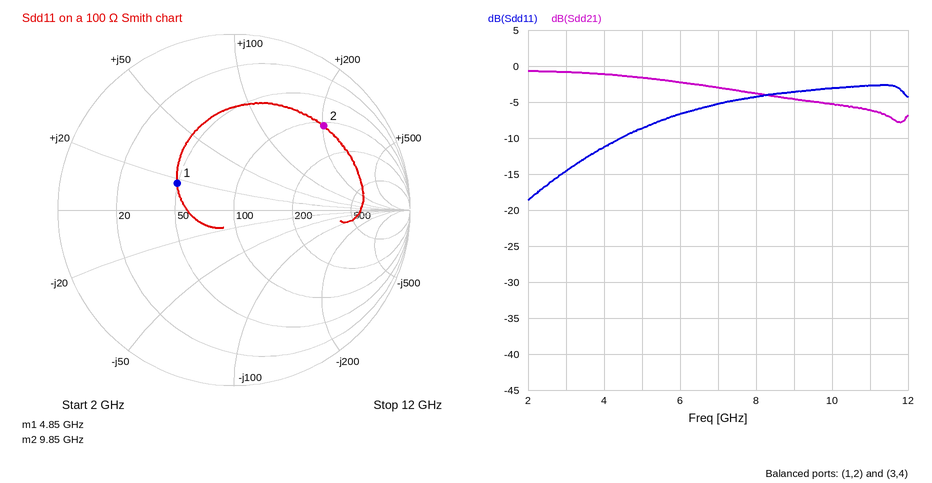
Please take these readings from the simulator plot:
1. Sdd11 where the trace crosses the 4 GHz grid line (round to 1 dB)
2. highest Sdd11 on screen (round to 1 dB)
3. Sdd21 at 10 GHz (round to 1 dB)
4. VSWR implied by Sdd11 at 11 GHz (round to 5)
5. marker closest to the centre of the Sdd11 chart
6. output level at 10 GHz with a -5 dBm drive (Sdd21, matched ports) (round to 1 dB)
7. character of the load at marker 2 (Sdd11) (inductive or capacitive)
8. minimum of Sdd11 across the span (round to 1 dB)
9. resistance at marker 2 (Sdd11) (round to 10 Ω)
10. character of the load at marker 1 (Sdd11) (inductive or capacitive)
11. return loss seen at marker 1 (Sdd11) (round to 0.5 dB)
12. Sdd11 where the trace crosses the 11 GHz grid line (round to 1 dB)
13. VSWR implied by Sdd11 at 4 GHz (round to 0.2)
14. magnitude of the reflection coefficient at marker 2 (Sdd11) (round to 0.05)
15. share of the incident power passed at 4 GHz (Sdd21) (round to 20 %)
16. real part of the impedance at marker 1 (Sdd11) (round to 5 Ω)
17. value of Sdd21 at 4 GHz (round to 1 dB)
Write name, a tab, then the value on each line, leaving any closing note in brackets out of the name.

Sdd11 where the trace crosses the 4 GHz grid line	-11 dB
highest Sdd11 on screen	-3 dB
Sdd21 at 10 GHz	-5 dB
VSWR implied by Sdd11 at 11 GHz	5
marker closest to the centre of the Sdd11 chart	marker 1
output level at 10 GHz with a -5 dBm drive (Sdd21, matched ports)	-10 dBm
character of the load at marker 2 (Sdd11)	inductive
minimum of Sdd11 across the span	-19 dB
resistance at marker 2 (Sdd11)	110 Ω
character of the load at marker 1 (Sdd11)	inductive
return loss seen at marker 1 (Sdd11)	9.0 dB
Sdd11 where the trace crosses the 11 GHz grid line	-3 dB
VSWR implied by Sdd11 at 4 GHz	1.8
magnitude of the reflection coefficient at marker 2 (Sdd11)	0.70
share of the incident power passed at 4 GHz (Sdd21)	80 %
real part of the impedance at marker 1 (Sdd11)	50 Ω
value of Sdd21 at 4 GHz	-1 dB
